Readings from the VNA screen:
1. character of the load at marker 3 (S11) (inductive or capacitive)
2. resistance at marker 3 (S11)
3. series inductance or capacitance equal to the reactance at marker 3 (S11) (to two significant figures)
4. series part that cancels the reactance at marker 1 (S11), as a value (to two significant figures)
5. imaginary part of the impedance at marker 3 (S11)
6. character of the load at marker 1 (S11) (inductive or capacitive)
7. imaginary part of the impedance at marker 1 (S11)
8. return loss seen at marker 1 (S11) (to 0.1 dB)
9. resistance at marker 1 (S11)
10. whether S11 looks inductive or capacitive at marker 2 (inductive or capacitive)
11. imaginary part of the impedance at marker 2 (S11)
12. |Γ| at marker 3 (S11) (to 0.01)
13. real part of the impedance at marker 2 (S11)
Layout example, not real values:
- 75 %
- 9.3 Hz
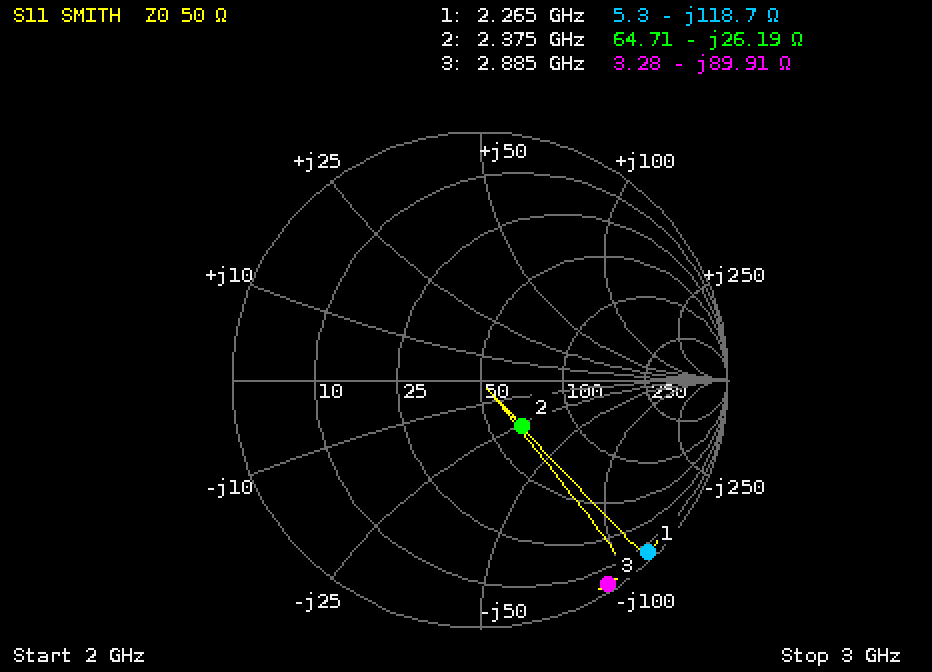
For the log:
- capacitive
- 3.28 Ω
- 610 fF
- 8.3 nH
- -89.91 Ω
- capacitive
- -118.7 Ω
- 0.3 dB
- 5.3 Ω
- capacitive
- -26.19 Ω
- 0.97
- 64.71 Ω
